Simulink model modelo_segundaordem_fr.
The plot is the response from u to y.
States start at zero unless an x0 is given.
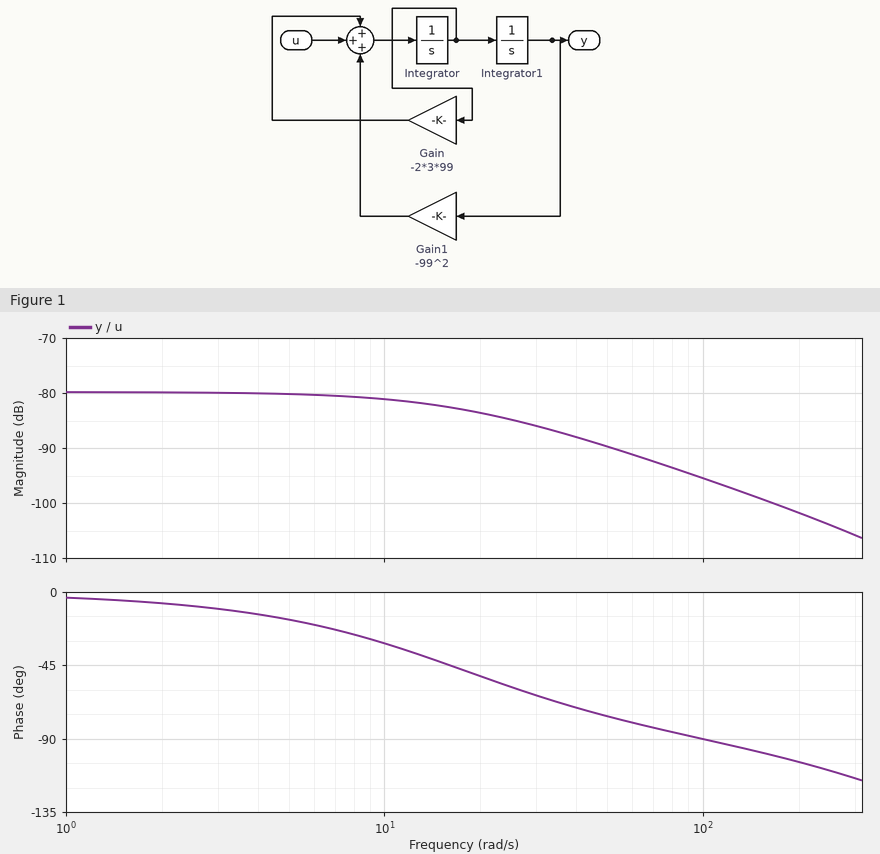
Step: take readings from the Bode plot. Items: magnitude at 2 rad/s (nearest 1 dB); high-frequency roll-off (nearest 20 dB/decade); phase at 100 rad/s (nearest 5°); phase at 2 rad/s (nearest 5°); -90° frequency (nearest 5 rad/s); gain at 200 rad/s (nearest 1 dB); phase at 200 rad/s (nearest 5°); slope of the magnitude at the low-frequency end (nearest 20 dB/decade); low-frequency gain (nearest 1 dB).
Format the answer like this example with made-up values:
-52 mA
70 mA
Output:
-80 dB
-20 dB/decade
-90°
-5°
100 rad/s
-102 dB
-105°
0 dB/decade
-80 dB
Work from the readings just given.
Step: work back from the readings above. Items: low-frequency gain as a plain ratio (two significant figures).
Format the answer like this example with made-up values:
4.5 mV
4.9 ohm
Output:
0.00010
